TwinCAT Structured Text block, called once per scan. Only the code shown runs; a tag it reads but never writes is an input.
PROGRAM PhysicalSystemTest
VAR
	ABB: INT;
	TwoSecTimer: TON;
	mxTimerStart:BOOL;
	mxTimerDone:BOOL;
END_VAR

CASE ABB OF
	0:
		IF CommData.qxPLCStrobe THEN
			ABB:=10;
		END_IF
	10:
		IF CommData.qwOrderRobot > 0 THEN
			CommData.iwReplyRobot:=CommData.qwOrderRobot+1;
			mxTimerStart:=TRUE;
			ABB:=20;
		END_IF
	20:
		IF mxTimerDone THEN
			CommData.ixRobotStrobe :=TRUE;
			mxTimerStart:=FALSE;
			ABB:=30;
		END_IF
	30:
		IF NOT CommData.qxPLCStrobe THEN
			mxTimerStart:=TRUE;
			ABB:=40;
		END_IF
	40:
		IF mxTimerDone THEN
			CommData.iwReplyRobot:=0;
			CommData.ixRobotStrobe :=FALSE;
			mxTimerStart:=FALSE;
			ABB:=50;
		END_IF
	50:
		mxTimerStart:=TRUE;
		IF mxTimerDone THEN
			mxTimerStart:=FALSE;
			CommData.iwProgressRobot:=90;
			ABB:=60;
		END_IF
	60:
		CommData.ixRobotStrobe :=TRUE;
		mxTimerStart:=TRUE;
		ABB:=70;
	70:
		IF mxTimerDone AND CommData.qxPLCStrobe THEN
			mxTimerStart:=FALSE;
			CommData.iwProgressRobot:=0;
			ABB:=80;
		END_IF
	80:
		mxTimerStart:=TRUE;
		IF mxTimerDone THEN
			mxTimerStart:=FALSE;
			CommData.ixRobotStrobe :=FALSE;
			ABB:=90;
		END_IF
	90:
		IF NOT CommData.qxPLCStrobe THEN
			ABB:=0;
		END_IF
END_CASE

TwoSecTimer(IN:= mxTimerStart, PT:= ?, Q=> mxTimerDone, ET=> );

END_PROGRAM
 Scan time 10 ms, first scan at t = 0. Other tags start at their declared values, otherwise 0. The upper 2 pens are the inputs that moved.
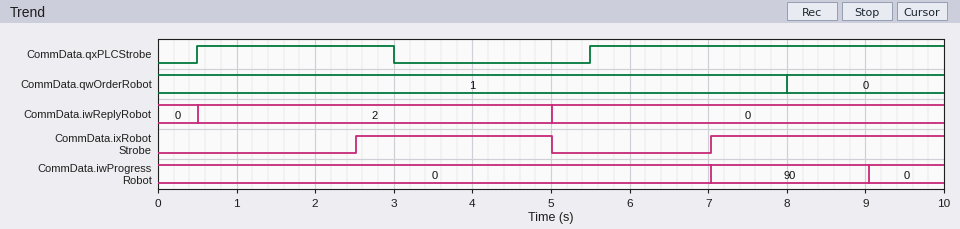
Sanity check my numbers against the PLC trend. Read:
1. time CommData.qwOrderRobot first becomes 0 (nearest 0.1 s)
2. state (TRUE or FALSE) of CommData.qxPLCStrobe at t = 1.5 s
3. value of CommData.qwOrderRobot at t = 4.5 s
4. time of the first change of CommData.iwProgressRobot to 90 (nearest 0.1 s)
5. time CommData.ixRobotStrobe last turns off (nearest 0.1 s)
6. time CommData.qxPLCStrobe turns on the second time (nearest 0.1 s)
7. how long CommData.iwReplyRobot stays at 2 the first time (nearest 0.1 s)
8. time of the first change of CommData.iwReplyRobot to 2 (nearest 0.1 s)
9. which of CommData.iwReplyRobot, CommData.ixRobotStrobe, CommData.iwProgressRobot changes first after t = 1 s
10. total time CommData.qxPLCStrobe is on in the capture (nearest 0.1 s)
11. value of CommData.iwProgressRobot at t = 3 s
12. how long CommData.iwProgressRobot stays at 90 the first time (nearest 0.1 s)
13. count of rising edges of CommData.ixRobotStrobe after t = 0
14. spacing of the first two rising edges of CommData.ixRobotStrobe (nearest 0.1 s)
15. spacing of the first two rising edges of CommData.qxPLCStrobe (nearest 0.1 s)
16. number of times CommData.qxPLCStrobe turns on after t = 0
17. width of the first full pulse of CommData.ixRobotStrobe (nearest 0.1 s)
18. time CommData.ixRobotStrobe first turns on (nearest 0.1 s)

8.0 s
TRUE
1
7.0 s
5.0 s
5.5 s
4.5 s
0.5 s
CommData.ixRobotStrobe
7.0 s
0
2.0 s
2
4.5 s
5.0 s
2
2.5 s
2.5 s
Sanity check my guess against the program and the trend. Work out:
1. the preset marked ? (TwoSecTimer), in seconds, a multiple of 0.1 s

2.0 s
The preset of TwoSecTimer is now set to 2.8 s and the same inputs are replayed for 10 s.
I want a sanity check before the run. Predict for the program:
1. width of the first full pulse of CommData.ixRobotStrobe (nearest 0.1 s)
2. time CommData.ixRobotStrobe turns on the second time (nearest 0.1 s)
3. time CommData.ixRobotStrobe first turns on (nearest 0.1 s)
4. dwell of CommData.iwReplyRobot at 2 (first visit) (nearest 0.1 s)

2.8 s
9.0 s
3.3 s
5.6 s
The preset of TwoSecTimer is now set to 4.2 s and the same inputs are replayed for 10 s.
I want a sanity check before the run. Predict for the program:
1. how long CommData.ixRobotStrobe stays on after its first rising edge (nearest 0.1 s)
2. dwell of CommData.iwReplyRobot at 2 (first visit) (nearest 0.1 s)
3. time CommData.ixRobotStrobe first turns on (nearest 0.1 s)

4.2 s
8.4 s
4.7 s
